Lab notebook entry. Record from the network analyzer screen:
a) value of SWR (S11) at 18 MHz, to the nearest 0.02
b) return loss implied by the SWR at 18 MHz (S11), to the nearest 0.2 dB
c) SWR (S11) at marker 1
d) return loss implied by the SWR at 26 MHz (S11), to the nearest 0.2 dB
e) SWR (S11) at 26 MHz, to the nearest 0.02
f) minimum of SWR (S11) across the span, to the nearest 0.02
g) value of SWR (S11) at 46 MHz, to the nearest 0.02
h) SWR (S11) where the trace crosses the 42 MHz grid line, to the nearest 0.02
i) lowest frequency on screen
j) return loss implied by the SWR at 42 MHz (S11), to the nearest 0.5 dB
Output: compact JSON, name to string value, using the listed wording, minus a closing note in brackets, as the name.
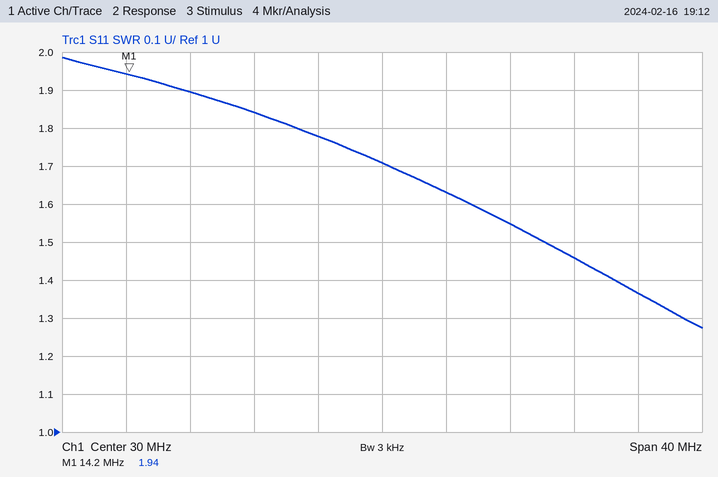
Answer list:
{"value of SWR (S11) at 18 MHz, to the nearest 0.02": "1.90", "return loss implied by the SWR at 18 MHz (S11), to the nearest 0.2 dB": "10.2 dB", "SWR (S11) at marker 1": "1.94", "return loss implied by the SWR at 26 MHz (S11), to the nearest 0.2 dB": "11.0 dB", "SWR (S11) at 26 MHz, to the nearest 0.02": "1.78", "minimum of SWR (S11) across the span, to the nearest 0.02": "1.28", "value of SWR (S11) at 46 MHz, to the nearest 0.02": "1.36", "SWR (S11) where the trace crosses the 42 MHz grid line, to the nearest 0.02": "1.46", "lowest frequency on screen": "10 MHz", "return loss implied by the SWR at 42 MHz (S11), to the nearest 0.5 dB": "14.5 dB"}
